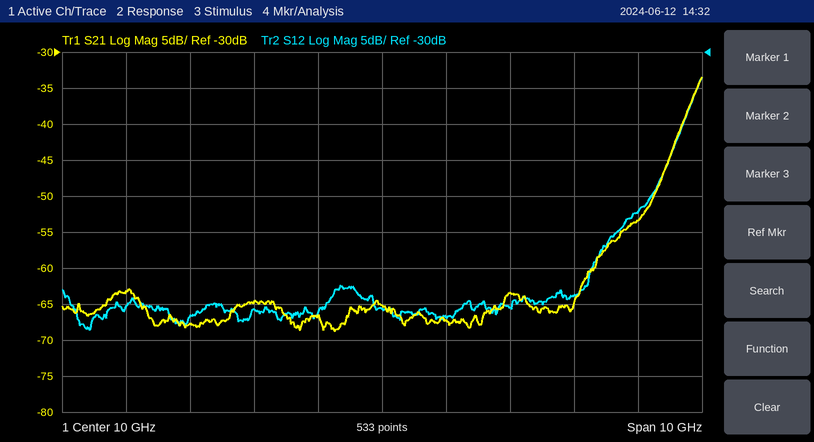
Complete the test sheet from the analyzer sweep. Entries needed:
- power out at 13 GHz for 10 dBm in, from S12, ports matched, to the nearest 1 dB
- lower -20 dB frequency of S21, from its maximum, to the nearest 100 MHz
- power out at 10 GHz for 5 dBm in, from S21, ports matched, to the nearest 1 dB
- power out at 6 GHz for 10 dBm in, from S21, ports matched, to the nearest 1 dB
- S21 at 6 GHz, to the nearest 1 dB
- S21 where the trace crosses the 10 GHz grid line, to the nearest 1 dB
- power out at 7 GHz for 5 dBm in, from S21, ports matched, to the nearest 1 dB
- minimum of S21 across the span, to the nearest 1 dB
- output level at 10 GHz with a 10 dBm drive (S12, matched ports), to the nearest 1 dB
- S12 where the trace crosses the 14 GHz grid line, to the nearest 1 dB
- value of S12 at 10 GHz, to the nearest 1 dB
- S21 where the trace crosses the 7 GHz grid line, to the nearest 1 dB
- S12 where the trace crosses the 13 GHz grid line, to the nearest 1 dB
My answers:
-54 dBm
14.0 GHz
-60 dBm
-53 dBm
-63 dB
-65 dB
-63 dBm
-69 dB
-56 dBm
-52 dB
-66 dB
-68 dB
-64 dB
